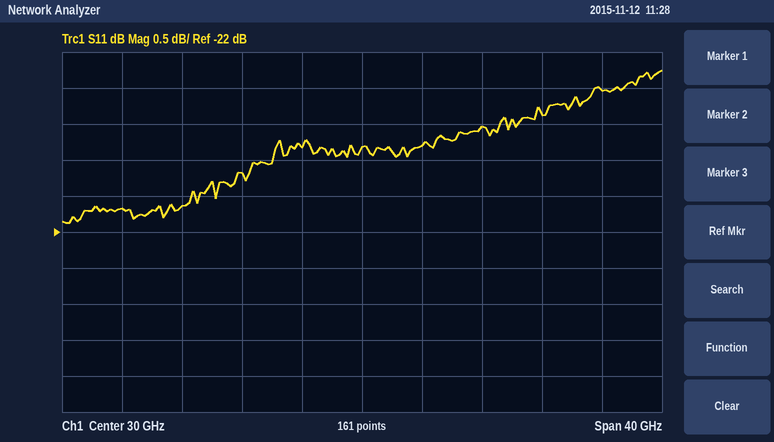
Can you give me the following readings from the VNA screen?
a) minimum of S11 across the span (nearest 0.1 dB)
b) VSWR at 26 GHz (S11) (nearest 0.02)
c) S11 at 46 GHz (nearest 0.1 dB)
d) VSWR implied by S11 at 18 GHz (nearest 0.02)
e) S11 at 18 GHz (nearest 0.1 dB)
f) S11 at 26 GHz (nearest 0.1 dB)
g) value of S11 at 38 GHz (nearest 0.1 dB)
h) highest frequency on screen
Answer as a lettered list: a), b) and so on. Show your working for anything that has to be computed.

a) -21.9 dB
b) |Γ| = 10^(-20.8/20) = 0.0912; VSWR = (1 + 0.0912)/(1 − 0.0912) ≈ 1.20
c) -20.0 dB
d) |Γ| = 10^(-21.6/20) = 0.0832; VSWR = (1 + 0.0832)/(1 − 0.0832) ≈ 1.18
e) -21.6 dB
f) -20.8 dB
g) -20.5 dB
h) 50 GHz
